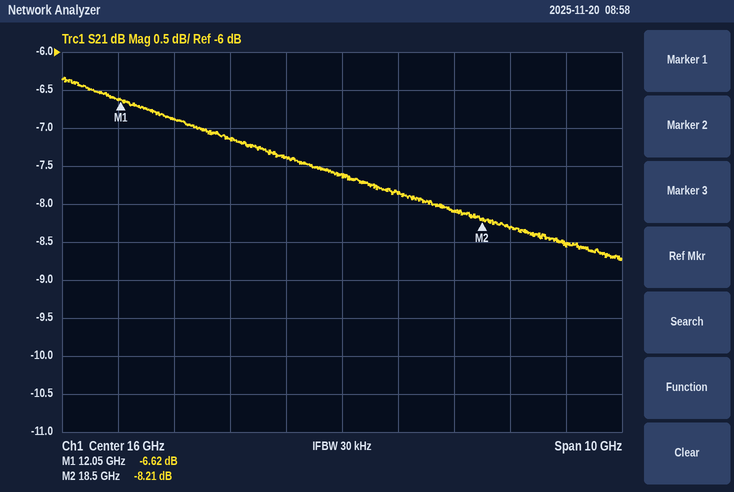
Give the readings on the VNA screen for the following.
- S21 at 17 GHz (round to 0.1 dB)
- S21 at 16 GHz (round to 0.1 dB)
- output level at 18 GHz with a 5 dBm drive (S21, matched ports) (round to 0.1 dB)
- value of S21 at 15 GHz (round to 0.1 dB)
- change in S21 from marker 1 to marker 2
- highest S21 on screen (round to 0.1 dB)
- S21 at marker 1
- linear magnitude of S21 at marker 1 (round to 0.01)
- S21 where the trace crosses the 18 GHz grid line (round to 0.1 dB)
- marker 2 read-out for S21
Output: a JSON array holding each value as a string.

["-7.9 dB", "-7.6 dB", "-3.1 dBm", "-7.4 dB", "-1.59 dB", "-6.3 dB", "-6.62 dB", "0.47", "-8.1 dB", "-8.21 dB"]
